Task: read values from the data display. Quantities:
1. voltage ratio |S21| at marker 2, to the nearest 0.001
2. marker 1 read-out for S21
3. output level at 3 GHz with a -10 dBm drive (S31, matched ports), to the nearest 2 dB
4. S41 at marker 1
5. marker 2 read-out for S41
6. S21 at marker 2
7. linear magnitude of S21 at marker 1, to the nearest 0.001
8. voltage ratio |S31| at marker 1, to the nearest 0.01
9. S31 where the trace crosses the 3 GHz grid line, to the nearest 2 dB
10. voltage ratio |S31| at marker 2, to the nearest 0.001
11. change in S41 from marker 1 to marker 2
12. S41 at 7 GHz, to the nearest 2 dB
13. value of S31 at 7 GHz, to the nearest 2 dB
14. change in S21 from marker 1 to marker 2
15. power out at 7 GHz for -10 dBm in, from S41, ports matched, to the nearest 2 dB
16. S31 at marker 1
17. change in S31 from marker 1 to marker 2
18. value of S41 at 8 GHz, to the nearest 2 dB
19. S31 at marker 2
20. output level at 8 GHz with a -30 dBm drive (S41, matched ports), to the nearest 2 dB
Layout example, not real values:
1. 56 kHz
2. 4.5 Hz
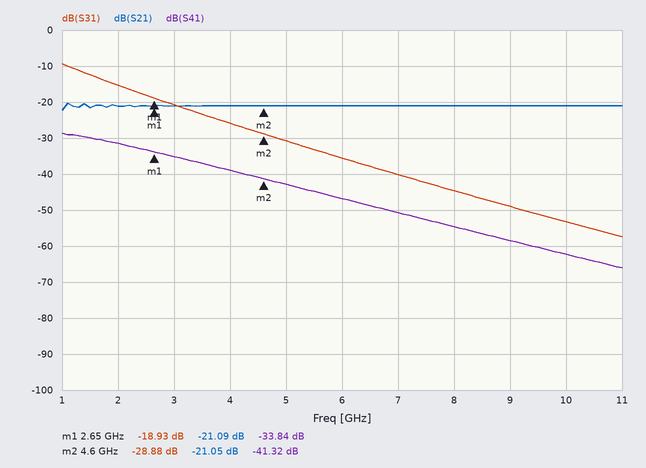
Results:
1. 0.089
2. -21.09 dB
3. -30 dBm
4. -33.84 dB
5. -41.32 dB
6. -21.05 dB
7. 0.088
8. 0.11
9. -20 dB
10. 0.036
11. -7.48 dB
12. -50 dB
13. -40 dB
14. 0.04 dB
15. -60 dBm
16. -18.93 dB
17. -9.95 dB
18. -54 dB
19. -28.88 dB
20. -84 dBm
